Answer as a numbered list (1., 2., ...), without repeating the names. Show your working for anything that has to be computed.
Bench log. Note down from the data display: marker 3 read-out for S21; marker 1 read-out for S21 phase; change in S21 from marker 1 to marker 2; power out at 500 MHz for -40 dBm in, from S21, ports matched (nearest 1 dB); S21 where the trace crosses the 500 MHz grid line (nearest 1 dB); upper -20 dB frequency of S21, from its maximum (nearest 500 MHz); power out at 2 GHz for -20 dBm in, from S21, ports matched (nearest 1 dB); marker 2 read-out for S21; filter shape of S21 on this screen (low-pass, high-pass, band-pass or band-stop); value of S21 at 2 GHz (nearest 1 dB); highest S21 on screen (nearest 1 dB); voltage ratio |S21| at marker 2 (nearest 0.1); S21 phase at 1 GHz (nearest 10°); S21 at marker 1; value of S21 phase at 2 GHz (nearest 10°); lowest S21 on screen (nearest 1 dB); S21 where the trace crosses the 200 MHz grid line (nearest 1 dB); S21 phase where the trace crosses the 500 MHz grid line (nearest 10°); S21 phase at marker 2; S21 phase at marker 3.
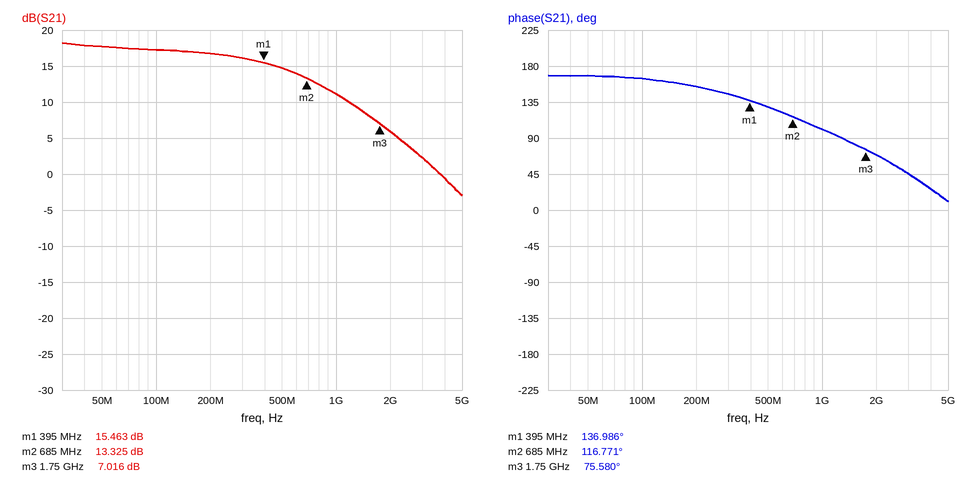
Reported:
1. 7.016 dB
2. 136.986°
3. 13.325 − (15.463) = -2.138 dB
4. -40 dBm + (15 dB) = -25 dBm
5. 15 dB
6. 4.5 GHz
7. -20 dBm + (6 dB) = -14 dBm
8. 13.325 dB
9. low-pass
10. 6 dB
11. 18 dB
12. 10^(13.325/20) ≈ 4.6
13. 100°
14. 15.463 dB
15. 70°
16. -3 dB
17. 17 dB
18. 130°
19. 116.771°
20. 75.580°
